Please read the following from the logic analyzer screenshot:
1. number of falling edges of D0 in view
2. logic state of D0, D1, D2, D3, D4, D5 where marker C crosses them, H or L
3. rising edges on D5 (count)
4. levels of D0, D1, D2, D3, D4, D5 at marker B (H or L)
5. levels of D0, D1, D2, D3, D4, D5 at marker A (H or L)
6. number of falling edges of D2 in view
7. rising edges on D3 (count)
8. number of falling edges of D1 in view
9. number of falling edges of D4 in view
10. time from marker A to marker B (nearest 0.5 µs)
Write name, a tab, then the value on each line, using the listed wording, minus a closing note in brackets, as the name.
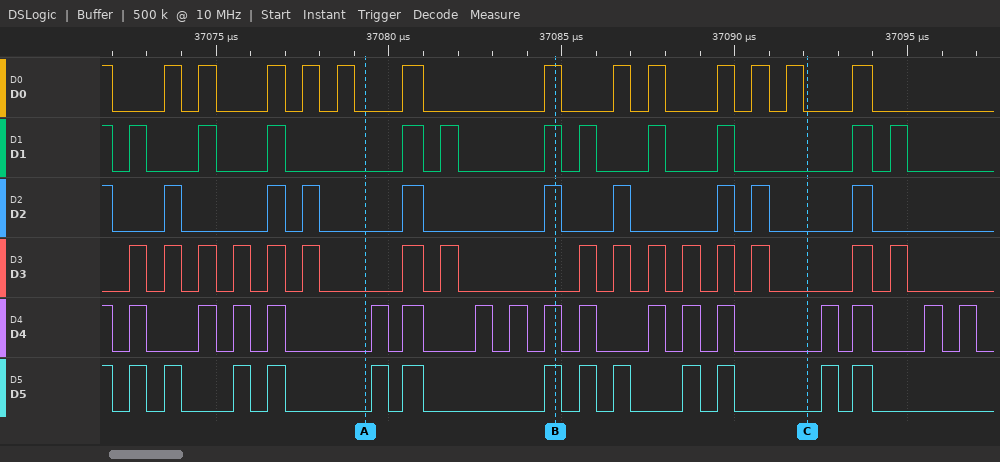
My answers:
number of falling edges of D0 in view	14
logic state of D0, D1, D2, D3, D4, D5 where marker C crosses them, H or L	D0=L, D1=L, D2=L, D3=L, D4=L, D5=L
rising edges on D5	13
levels of D0, D1, D2, D3, D4, D5 at marker B	D0=H, D1=H, D2=H, D3=L, D4=H, D5=H
levels of D0, D1, D2, D3, D4, D5 at marker A	D0=L, D1=L, D2=L, D3=L, D4=L, D5=L
number of falling edges of D2 in view	10
rising edges on D3	16
number of falling edges of D1 in view	12
number of falling edges of D4 in view	18
time from marker A to marker B	5.5 µs
